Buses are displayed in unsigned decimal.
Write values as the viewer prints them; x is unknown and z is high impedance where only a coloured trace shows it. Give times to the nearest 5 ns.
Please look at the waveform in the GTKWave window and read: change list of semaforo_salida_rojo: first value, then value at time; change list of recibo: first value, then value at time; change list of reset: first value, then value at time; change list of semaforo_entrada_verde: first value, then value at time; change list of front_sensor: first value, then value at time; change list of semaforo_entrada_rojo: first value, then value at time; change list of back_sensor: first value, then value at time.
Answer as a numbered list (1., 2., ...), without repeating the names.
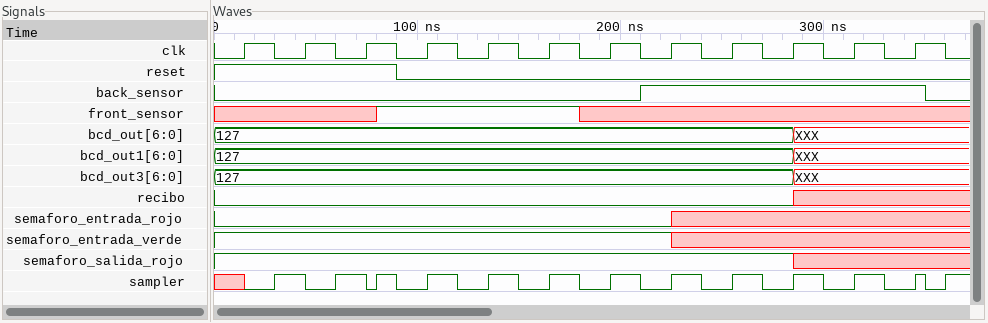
1. 1, x at 285 ns
2. 0, x at 285 ns
3. 1, 0 at 90 ns
4. 1, x at 225 ns
5. x, 1 at 80 ns, x at 180 ns
6. 0, x at 225 ns
7. 0, 1 at 210 ns, 0 at 350 ns
